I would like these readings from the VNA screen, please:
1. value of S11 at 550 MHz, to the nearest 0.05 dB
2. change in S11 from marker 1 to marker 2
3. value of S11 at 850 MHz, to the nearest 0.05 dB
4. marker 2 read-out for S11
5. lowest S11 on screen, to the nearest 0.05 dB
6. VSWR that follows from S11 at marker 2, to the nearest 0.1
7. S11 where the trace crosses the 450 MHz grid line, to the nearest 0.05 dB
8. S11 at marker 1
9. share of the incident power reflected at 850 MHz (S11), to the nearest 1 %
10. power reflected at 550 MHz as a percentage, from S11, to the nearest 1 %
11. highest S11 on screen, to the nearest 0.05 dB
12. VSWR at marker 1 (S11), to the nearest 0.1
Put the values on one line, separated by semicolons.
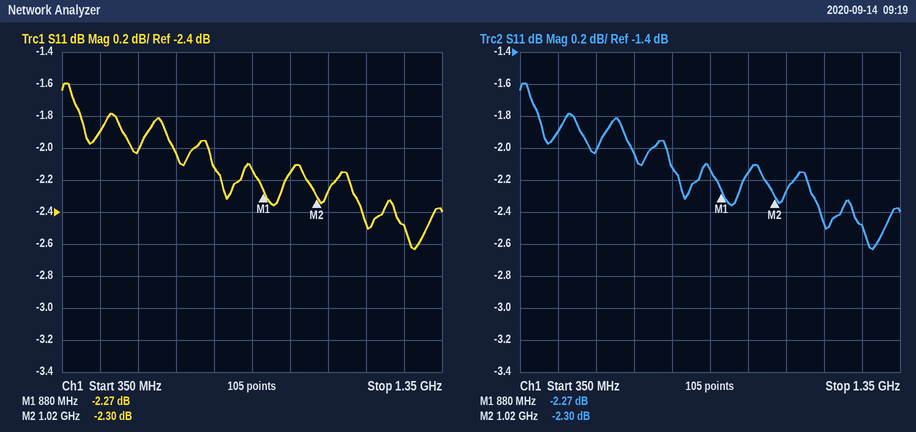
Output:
-2.00 dB; -0.03 dB; -2.15 dB; -2.30 dB; -2.65 dB; 7.6; -1.90 dB; -2.27 dB; 61 %; 63 %; -1.60 dB; 7.7
